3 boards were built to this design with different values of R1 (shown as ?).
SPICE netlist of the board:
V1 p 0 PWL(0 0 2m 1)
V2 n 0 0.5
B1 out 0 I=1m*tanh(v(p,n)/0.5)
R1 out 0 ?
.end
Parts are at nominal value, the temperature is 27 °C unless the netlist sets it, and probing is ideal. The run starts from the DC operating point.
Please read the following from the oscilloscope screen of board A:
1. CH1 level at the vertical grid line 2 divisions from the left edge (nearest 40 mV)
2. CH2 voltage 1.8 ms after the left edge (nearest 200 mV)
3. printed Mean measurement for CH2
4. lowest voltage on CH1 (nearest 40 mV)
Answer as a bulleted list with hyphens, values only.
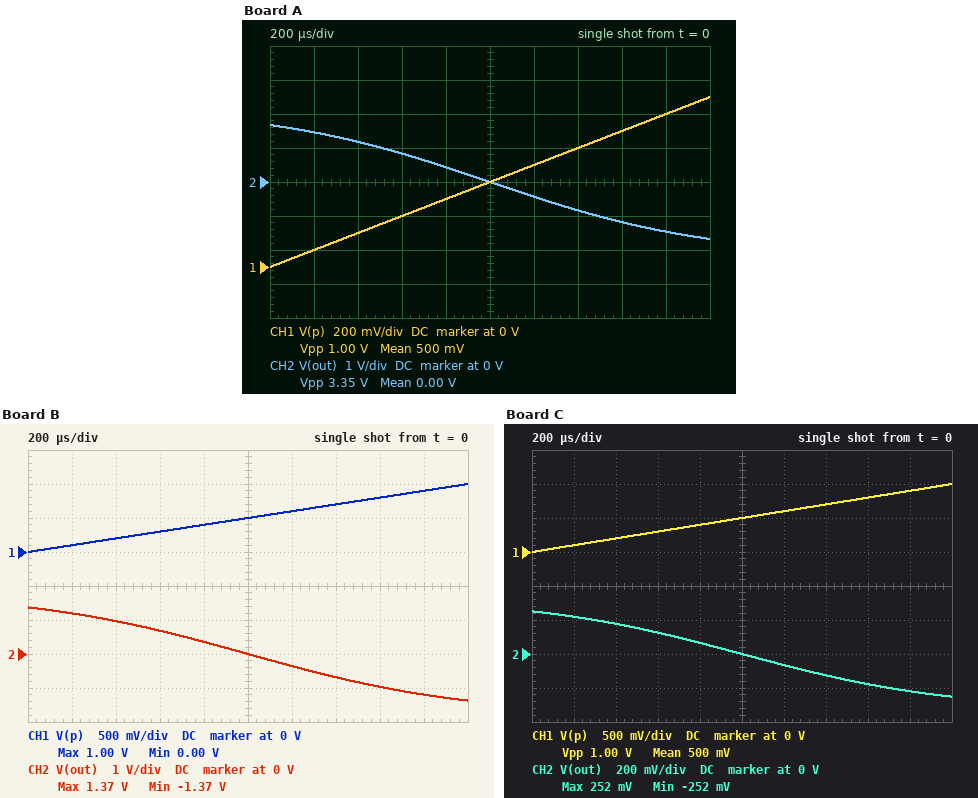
- 200 mV
- -1.4 V
- 0.00 V
- 0 V
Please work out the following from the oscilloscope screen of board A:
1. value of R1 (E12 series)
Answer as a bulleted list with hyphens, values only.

- 2.2 kΩ
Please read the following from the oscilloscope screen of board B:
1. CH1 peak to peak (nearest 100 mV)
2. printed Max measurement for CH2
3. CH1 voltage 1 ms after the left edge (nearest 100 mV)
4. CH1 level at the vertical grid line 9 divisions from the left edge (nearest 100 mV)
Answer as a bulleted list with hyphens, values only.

- 1.0 V
- 1.37 V
- 500 mV
- 900 mV
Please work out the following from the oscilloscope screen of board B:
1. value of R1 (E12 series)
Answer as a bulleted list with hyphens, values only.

- 1.8 kΩ
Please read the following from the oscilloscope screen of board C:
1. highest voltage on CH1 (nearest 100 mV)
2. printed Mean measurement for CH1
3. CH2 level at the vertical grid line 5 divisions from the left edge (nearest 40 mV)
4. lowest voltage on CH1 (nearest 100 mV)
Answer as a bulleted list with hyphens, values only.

- 1.0 V
- 500 mV
- 0 V
- 0 V
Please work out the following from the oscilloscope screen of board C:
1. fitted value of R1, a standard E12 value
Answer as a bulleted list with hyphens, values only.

- 330 Ω
